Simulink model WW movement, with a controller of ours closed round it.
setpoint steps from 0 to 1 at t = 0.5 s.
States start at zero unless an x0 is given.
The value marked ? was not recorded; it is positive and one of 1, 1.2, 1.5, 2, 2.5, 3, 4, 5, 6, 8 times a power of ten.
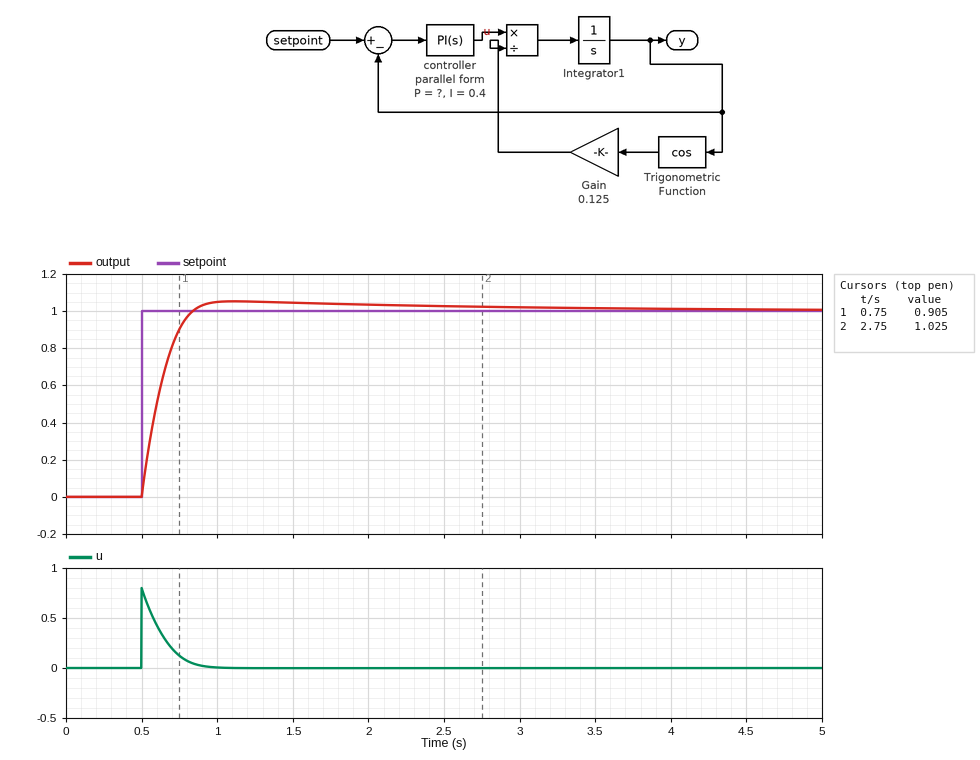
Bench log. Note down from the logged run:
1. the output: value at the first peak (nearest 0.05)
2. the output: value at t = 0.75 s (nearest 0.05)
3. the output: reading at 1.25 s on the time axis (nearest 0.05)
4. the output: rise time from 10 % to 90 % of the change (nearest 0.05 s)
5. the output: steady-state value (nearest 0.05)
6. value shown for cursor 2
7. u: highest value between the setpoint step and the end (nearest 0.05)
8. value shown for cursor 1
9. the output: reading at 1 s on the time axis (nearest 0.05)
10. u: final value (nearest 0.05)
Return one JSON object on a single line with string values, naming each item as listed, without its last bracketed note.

{"the output: value at the first peak": "1.05", "the output: value at t = 0.75 s": "0.90", "the output: reading at 1.25 s on the time axis": "1.05", "the output: rise time from 10 % to 90 % of the change": "0.25 s", "the output: steady-state value": "1.00", "value shown for cursor 2": "1.025", "u: highest value between the setpoint step and the end": "0.80", "value shown for cursor 1": "0.905", "the output: reading at 1 s on the time axis": "1.05", "u: final value": "0.00"}
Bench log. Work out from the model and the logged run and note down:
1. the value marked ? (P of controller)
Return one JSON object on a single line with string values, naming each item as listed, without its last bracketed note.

{"the value marked ?": "0.8"}
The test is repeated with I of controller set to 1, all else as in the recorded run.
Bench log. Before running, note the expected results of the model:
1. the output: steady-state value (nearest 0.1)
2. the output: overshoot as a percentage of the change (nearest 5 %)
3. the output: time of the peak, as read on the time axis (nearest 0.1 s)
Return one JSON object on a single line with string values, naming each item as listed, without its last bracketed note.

{"the output: steady-state value": "1.0", "the output: overshoot as a percentage of the change": "10 %", "the output: time of the peak, as read on the time axis": "1.0 s"}
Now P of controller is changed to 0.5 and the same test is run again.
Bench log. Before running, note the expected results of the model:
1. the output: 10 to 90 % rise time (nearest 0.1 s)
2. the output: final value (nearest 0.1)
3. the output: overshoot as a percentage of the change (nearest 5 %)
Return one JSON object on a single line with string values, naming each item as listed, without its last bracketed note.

{"the output: 10 to 90 % rise time": "0.3 s", "the output: final value": "1.0", "the output: overshoot as a percentage of the change": "10 %"}
